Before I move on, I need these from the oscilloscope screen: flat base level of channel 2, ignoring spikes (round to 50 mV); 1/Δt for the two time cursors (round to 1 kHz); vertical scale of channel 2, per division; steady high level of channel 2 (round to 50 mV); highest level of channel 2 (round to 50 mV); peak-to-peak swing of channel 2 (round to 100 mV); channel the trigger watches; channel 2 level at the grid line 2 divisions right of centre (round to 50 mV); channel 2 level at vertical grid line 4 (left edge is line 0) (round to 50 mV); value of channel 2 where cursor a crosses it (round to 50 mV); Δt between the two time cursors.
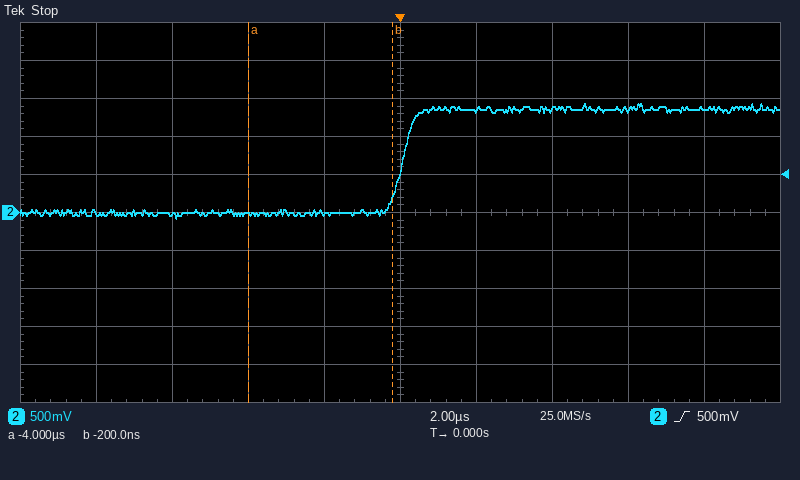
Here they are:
0 mV
263 kHz
500 mV
1.35 V
1.45 V
1.50 V
channel 2
1.35 V
0 mV
0 mV
3.8 µs
